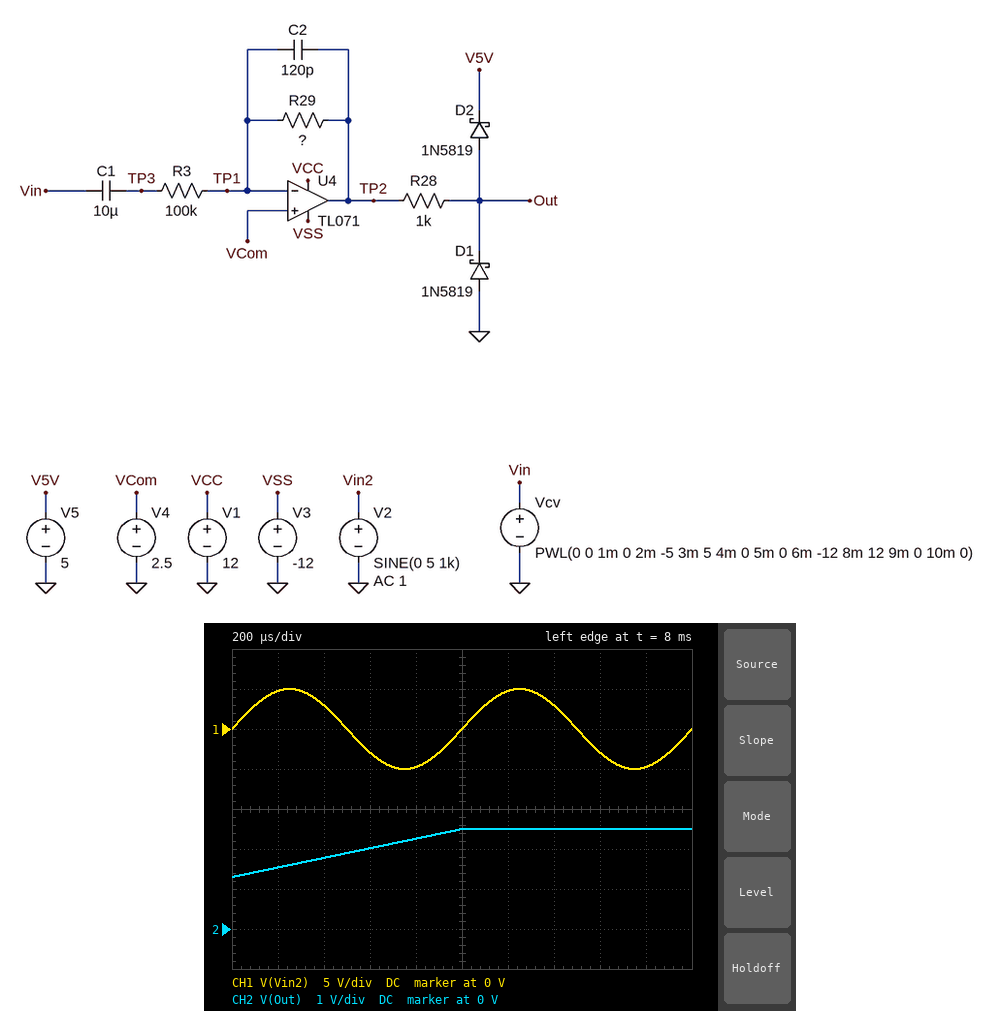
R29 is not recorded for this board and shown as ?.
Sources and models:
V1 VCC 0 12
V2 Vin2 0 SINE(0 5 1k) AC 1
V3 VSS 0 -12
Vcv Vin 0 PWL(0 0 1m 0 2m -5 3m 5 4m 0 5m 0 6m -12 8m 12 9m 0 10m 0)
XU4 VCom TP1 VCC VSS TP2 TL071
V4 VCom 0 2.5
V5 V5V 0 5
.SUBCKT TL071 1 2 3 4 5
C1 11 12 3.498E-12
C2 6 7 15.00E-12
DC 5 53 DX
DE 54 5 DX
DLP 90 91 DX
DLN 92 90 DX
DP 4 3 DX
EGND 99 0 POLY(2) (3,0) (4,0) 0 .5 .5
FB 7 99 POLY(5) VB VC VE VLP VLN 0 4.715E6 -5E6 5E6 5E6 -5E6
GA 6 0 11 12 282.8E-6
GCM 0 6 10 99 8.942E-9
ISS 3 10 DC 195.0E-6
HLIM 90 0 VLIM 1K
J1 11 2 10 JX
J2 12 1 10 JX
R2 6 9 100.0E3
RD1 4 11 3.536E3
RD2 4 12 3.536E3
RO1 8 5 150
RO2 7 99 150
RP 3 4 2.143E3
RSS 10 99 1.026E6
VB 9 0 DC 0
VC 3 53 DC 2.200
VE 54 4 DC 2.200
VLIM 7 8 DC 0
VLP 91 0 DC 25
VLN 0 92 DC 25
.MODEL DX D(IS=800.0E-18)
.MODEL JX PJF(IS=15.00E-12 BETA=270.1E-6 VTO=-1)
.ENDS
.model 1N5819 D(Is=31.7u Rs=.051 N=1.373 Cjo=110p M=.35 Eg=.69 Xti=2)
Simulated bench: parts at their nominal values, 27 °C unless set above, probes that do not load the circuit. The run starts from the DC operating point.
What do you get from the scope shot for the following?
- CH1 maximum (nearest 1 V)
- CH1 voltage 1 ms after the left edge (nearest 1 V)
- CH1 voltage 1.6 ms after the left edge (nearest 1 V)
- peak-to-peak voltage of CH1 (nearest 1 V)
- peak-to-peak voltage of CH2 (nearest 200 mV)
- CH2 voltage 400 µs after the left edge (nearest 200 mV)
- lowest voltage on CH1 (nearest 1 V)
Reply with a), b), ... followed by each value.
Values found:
a) 5 V
b) 0 V
c) -3 V
d) 10 V
e) 1.2 V
f) 1.8 V
g) -5 V
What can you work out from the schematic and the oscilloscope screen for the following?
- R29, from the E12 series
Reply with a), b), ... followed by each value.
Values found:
a) 10 kΩ
